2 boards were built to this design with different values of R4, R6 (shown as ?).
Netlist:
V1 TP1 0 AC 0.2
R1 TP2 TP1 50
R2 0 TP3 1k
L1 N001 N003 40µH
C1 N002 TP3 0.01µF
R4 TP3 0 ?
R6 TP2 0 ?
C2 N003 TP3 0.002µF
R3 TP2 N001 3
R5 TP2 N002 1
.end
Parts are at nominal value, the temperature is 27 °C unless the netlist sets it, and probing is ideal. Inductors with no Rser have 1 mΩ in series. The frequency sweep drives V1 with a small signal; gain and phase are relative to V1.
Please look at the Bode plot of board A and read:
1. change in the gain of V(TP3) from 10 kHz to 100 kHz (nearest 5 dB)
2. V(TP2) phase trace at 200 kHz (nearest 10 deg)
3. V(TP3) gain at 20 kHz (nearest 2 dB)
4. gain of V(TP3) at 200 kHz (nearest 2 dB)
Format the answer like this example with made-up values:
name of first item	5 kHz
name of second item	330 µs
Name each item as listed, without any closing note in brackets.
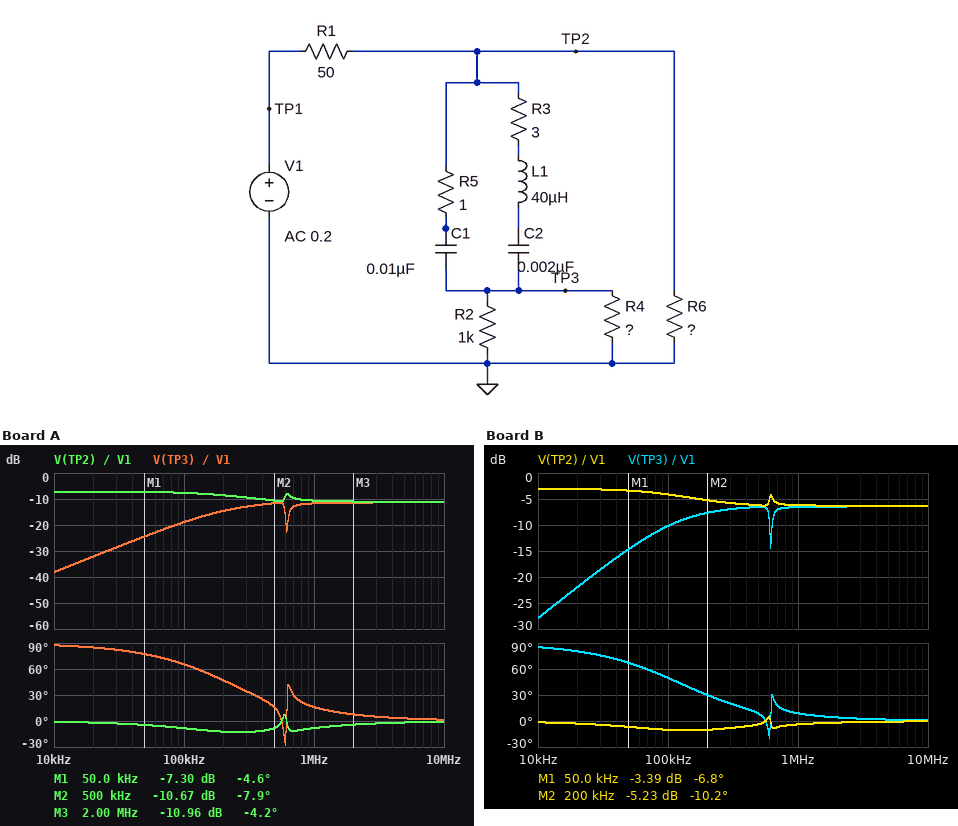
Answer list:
change in the gain of V(TP3) from 10 kHz to 100 kHz	20 dB
V(TP2) phase trace at 200 kHz	-10 deg
V(TP3) gain at 20 kHz	-32 dB
gain of V(TP3) at 200 kHz	-14 dB
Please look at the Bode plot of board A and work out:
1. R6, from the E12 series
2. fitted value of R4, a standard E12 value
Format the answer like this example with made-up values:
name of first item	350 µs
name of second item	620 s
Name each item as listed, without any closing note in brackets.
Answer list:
R6, from the E12 series	39 Ω
fitted value of R4, a standard E12 value	39 Ω
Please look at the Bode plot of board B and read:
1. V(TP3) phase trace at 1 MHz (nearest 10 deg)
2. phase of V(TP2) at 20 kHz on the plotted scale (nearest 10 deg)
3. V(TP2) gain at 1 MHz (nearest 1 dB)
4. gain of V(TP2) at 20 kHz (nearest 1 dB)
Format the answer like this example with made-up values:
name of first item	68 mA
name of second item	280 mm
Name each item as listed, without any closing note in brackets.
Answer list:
V(TP3) phase trace at 1 MHz	10 deg
phase of V(TP2) at 20 kHz on the plotted scale	0 deg
V(TP2) gain at 1 MHz	-6 dB
gain of V(TP2) at 20 kHz	-3 dB
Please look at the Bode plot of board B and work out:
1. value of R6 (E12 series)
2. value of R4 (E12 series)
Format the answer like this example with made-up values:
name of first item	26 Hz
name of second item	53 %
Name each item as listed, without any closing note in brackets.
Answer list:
value of R6	120 Ω
value of R4	82 Ω
